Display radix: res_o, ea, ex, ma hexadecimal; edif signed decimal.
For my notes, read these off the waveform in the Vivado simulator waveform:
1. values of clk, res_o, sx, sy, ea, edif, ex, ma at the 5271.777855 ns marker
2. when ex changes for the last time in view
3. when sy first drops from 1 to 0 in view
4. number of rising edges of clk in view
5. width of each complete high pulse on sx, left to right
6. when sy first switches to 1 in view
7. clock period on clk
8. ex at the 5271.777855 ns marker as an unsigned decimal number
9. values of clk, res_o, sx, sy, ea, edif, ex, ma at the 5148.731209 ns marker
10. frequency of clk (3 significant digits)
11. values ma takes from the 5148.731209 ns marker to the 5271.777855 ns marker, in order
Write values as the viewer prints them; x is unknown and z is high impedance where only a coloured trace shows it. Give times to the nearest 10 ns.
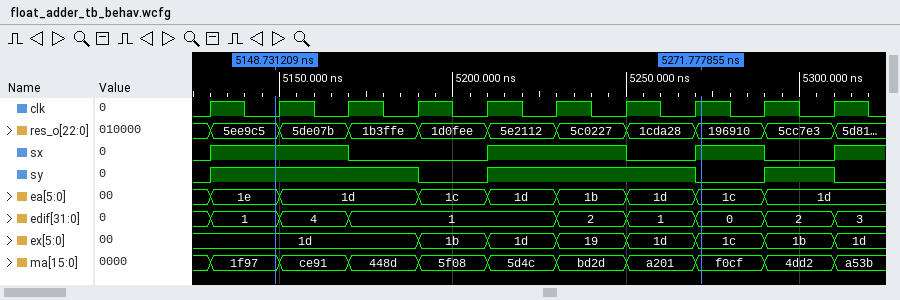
clk=1, res_o=196910, sx=1, sy=0, ea=1c, edif=0, ex=1c, ma=f0cf
5310 ns
5190 ns
10
40 ns, 40 ns, 20 ns
5130 ns
20 ns
28
clk=0, res_o=5ee9c5, sx=1, sy=1, ea=1e, edif=1, ex=1d, ma=1f97
50.0 MHz
1f97, ce91, 448d, 5f08, 5d4c, bd2d, a201, f0cf
